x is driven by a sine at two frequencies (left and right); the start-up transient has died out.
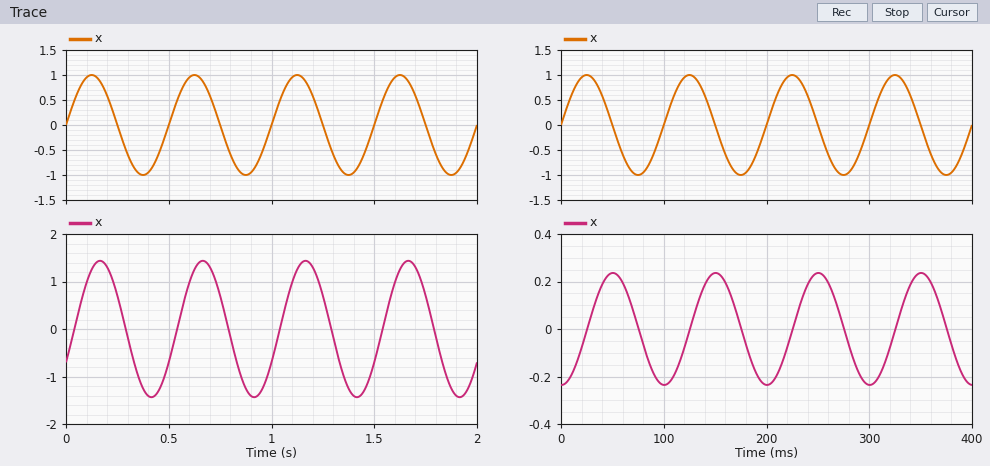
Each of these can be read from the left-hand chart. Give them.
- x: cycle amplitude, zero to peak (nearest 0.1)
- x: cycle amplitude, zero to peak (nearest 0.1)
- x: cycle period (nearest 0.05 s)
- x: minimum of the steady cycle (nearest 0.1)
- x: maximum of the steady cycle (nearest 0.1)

1.4
1.0
0.50 s
-1.4
1.4
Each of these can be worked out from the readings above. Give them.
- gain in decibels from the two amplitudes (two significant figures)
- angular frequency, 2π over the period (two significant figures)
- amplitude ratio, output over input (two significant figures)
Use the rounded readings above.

2.9 dB
13 rad/s
1.4
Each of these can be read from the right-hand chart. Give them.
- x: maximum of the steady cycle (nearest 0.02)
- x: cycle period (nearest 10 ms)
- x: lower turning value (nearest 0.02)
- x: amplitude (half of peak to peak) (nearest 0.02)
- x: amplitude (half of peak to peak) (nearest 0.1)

0.24
100 ms
-0.24
0.24
1.0
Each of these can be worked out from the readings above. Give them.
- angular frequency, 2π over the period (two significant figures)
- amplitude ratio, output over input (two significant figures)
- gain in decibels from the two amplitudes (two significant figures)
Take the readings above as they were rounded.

0.063 rad/ms
0.24
-12 dB
